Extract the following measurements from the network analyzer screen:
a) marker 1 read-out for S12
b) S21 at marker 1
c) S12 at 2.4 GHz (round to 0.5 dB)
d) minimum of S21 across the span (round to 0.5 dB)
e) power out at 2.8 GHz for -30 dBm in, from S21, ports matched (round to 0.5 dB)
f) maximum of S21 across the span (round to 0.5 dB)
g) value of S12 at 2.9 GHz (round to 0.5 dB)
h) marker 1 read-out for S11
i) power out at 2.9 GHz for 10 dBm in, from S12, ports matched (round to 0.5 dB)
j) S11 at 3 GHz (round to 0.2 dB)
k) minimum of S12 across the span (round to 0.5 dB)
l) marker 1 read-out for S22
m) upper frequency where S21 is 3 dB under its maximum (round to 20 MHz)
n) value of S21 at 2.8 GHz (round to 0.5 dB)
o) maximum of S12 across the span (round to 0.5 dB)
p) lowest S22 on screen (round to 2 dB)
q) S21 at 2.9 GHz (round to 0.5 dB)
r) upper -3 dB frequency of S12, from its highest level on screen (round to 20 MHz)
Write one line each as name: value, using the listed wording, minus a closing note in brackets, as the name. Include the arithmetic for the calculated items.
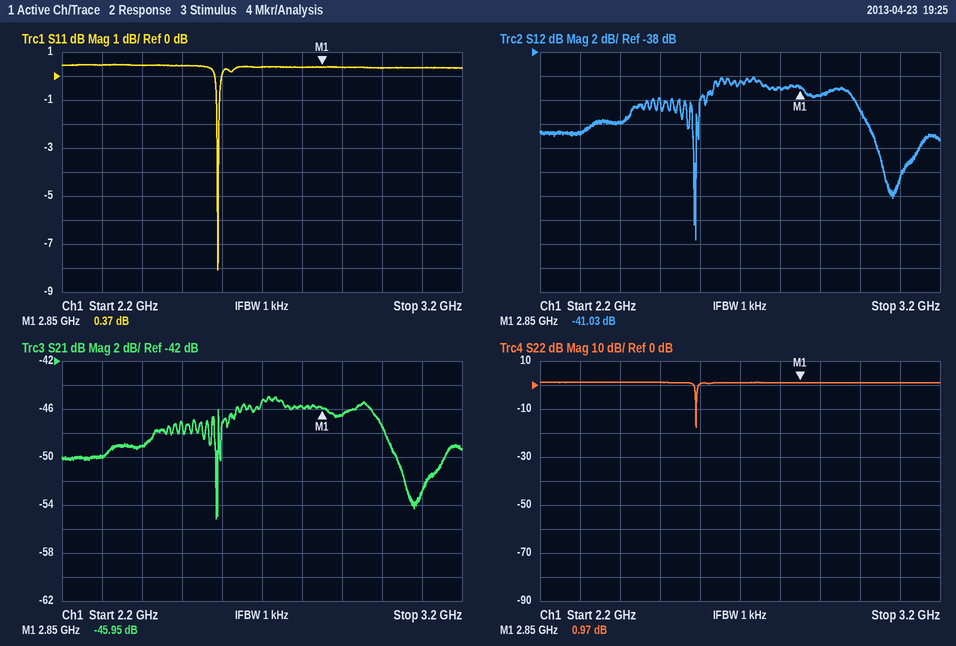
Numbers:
marker 1 read-out for S12: -41.03 dB
S21 at marker 1: -45.95 dB
S12 at 2.4 GHz: -44.0 dB
minimum of S21 across the span: -55.0 dB
power out at 2.8 GHz for -30 dBm in, from S21, ports matched: -30 dBm + (-46.0 dB) = -76.0 dBm
maximum of S21 across the span: -45.0 dB
value of S12 at 2.9 GHz: -41.5 dB
marker 1 read-out for S11: 0.37 dB
power out at 2.9 GHz for 10 dBm in, from S12, ports matched: 10 dBm + (-41.5 dB) = -31.5 dBm
S11 at 3 GHz: 0.4 dB
minimum of S12 across the span: -53.5 dB
marker 1 read-out for S22: 0.97 dB
upper frequency where S21 is 3 dB under its maximum: 3.00 GHz
value of S21 at 2.8 GHz: -46.0 dB
maximum of S12 across the span: -40.0 dB
lowest S22 on screen: -18 dB
S21 at 2.9 GHz: -46.5 dB
upper -3 dB frequency of S12, from its highest level on screen: 3.00 GHz
